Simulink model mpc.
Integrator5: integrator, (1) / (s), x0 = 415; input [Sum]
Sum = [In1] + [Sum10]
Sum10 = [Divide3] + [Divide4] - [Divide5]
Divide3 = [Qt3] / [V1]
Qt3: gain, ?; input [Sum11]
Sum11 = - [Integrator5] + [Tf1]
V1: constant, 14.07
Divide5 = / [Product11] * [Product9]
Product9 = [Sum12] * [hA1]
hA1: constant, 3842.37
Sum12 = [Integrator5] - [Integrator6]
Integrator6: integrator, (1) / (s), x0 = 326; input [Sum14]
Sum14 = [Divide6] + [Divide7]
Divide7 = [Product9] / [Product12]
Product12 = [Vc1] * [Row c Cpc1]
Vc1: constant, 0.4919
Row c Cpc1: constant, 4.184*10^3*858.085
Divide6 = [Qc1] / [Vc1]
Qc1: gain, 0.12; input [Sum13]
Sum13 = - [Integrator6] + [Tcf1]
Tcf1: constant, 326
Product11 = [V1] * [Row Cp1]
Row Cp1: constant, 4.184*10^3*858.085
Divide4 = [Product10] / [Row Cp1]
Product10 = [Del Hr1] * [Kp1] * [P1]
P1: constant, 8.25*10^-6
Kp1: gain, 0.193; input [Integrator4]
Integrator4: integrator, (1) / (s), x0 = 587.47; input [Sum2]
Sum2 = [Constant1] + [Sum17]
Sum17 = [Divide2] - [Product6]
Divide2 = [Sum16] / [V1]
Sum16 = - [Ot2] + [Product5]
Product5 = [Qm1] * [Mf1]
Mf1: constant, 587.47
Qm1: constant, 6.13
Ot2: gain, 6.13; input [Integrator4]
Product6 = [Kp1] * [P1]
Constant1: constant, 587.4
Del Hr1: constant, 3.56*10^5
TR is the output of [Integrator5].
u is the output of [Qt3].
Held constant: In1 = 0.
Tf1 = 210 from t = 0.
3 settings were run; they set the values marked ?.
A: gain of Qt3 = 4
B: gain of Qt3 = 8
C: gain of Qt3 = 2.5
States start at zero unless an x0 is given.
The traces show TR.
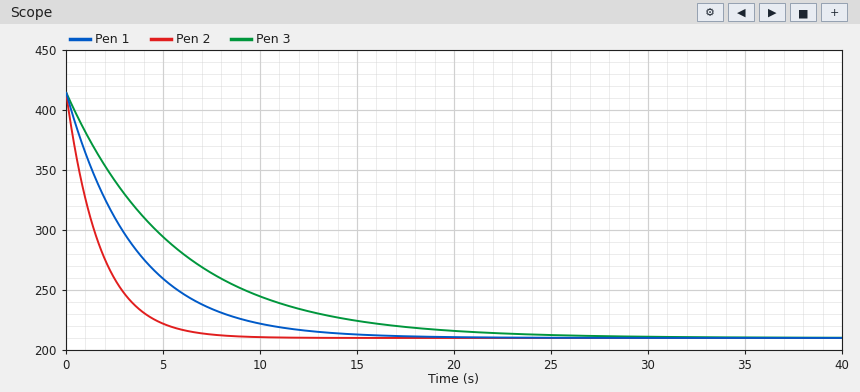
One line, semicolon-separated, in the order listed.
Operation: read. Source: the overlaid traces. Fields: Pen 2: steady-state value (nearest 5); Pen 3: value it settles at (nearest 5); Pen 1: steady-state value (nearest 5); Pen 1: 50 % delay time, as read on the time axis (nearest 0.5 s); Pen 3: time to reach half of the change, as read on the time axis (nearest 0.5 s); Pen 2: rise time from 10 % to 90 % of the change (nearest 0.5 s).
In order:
210; 210; 210; 2.5 s; 4.0 s; 4.0 s
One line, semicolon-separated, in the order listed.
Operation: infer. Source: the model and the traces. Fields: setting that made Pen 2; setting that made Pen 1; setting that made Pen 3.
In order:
B; A; C
